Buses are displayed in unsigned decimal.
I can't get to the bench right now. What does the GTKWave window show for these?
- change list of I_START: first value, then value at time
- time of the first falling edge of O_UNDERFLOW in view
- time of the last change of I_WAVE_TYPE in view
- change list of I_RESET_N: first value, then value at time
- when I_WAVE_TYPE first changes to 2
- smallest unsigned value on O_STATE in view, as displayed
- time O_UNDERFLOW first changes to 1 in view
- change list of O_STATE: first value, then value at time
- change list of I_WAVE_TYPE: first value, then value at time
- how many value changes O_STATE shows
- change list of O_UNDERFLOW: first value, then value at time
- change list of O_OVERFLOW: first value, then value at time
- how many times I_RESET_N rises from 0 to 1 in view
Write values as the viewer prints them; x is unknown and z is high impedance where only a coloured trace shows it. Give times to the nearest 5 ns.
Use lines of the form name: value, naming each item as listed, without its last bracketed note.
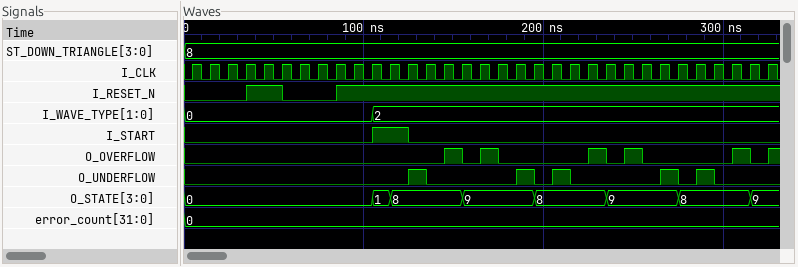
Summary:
change list of I_START: first value, then value at time: 0, 1 at 105 ns, 0 at 125 ns
time of the first falling edge of O_UNDERFLOW in view: 135 ns
time of the last change of I_WAVE_TYPE in view: 105 ns
change list of I_RESET_N: first value, then value at time: 0, 1 at 35 ns, 0 at 55 ns, 1 at 85 ns
when I_WAVE_TYPE first changes to 2: 105 ns
smallest unsigned value on O_STATE in view, as displayed: 0
time O_UNDERFLOW first changes to 1 in view: 125 ns
change list of O_STATE: first value, then value at time: 0, 1 at 105 ns, 8 at 115 ns, 9 at 155 ns, 8 at 195 ns, 9 at 235 ns, 8 at 275 ns, 9 at 315 ns
change list of I_WAVE_TYPE: first value, then value at time: 0, 2 at 105 ns
how many value changes O_STATE shows: 7
change list of O_UNDERFLOW: first value, then value at time: 0, 1 at 125 ns, 0 at 135 ns, 1 at 185 ns, 0 at 195 ns, 1 at 205 ns, 0 at 215 ns, 1 at 265 ns, 0 at 275 ns, 1 at 285 ns, 0 at 295 ns
change list of O_OVERFLOW: first value, then value at time: 0, 1 at 145 ns, 0 at 155 ns, 1 at 165 ns, 0 at 175 ns, 1 at 225 ns, 0 at 235 ns, 1 at 245 ns, 0 at 255 ns, 1 at 305 ns, 0 at 315 ns, 1 at 325 ns
how many times I_RESET_N rises from 0 to 1 in view: 2
